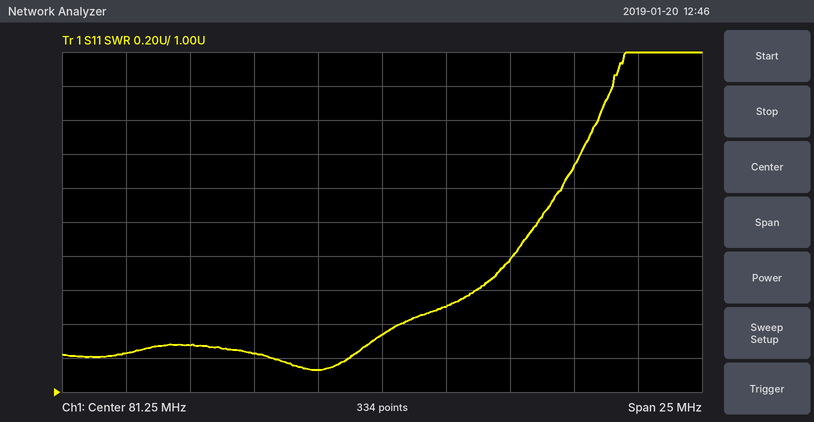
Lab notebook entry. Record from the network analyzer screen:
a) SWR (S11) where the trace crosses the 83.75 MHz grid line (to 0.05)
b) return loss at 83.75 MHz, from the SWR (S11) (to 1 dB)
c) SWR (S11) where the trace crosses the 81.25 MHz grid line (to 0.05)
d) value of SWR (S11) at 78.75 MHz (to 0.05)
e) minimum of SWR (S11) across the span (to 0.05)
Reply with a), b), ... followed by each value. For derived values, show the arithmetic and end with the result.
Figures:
a) 1.50
b) −20 log10((1.5 − 1)/(1.5 + 1)) ≈ 14 dB
c) 1.35
d) 1.15
e) 1.15
